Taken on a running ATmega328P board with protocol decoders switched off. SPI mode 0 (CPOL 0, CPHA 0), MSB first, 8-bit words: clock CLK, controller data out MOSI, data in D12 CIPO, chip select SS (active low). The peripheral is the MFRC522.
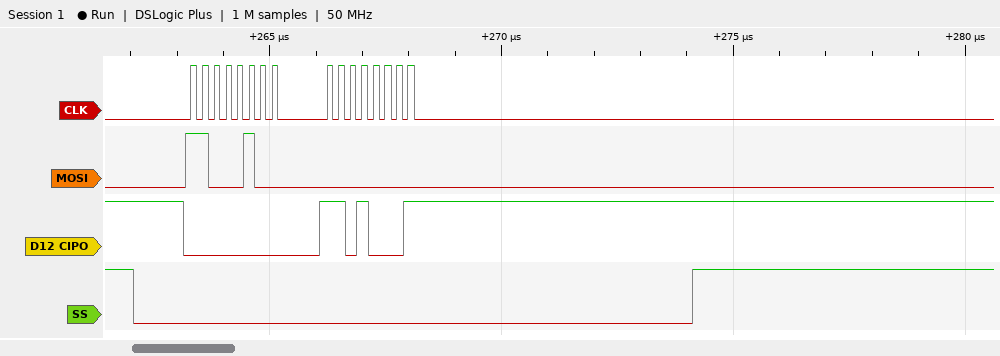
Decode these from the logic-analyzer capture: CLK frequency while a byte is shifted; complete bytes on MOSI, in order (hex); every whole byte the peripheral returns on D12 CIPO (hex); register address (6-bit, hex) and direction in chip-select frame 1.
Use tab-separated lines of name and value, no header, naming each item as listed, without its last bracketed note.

CLK frequency while a byte is shifted	4 MHz
complete bytes on MOSI, in order	C4 00
every whole byte the peripheral returns on D12 CIPO	00 D1
register address (6-bit, hex) and direction in chip-select frame 1	0x22 read
